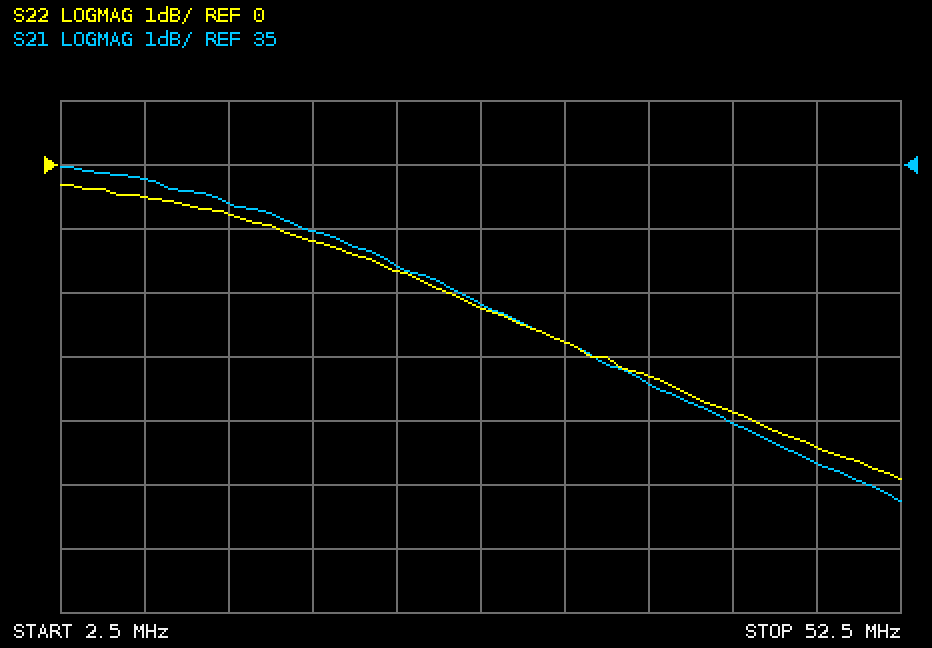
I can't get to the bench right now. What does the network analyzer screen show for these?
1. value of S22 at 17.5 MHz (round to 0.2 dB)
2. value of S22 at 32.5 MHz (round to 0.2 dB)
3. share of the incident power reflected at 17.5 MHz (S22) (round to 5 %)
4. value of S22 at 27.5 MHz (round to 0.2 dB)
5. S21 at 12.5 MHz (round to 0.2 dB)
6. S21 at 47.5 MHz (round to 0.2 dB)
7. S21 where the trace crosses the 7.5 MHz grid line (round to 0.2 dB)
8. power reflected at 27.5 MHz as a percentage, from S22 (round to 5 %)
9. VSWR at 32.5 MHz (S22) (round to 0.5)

-1.2 dB
-2.8 dB
75 %
-2.2 dB
34.4 dB
30.4 dB
34.8 dB
60 %
6.5
